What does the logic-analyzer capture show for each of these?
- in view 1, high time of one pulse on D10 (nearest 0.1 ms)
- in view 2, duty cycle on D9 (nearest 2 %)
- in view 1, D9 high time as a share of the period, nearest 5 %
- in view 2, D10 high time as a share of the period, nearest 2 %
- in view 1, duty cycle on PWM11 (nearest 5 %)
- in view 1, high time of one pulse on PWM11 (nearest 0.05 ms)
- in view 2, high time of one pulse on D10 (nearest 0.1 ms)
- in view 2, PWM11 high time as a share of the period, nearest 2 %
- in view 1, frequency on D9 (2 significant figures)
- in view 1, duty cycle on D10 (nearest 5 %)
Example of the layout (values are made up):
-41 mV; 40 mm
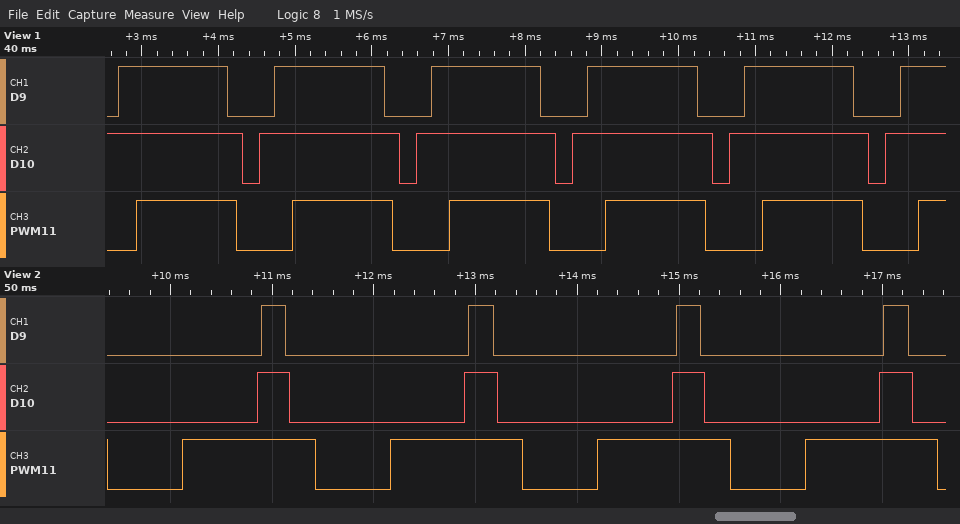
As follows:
1.8 ms; 12 %; 70 %; 16 %; 65 %; 1.30 ms; 0.3 ms; 64 %; 490 Hz; 90 %
